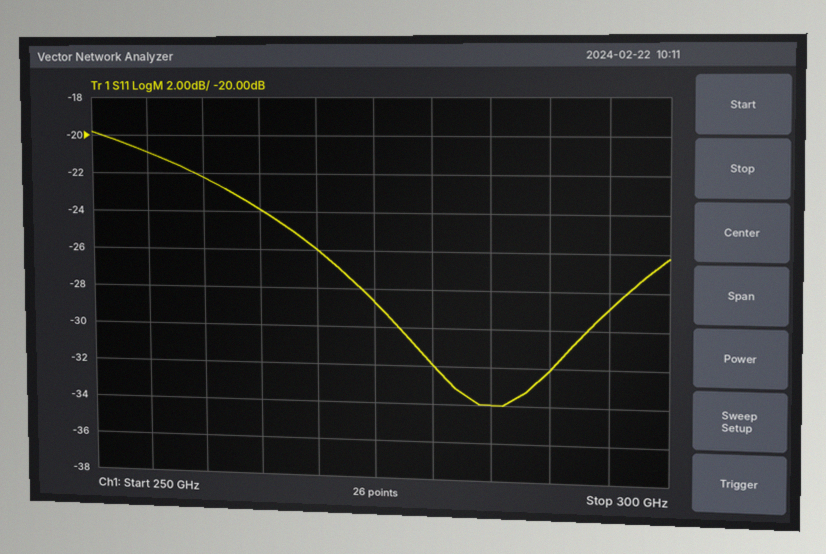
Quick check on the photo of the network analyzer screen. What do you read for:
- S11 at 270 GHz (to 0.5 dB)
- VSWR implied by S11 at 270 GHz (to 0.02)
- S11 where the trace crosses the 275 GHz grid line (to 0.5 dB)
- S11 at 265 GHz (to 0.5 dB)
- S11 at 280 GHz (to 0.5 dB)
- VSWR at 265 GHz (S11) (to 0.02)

-26.0 dB
1.10
-28.5 dB
-24.0 dB
-32.0 dB
1.14
